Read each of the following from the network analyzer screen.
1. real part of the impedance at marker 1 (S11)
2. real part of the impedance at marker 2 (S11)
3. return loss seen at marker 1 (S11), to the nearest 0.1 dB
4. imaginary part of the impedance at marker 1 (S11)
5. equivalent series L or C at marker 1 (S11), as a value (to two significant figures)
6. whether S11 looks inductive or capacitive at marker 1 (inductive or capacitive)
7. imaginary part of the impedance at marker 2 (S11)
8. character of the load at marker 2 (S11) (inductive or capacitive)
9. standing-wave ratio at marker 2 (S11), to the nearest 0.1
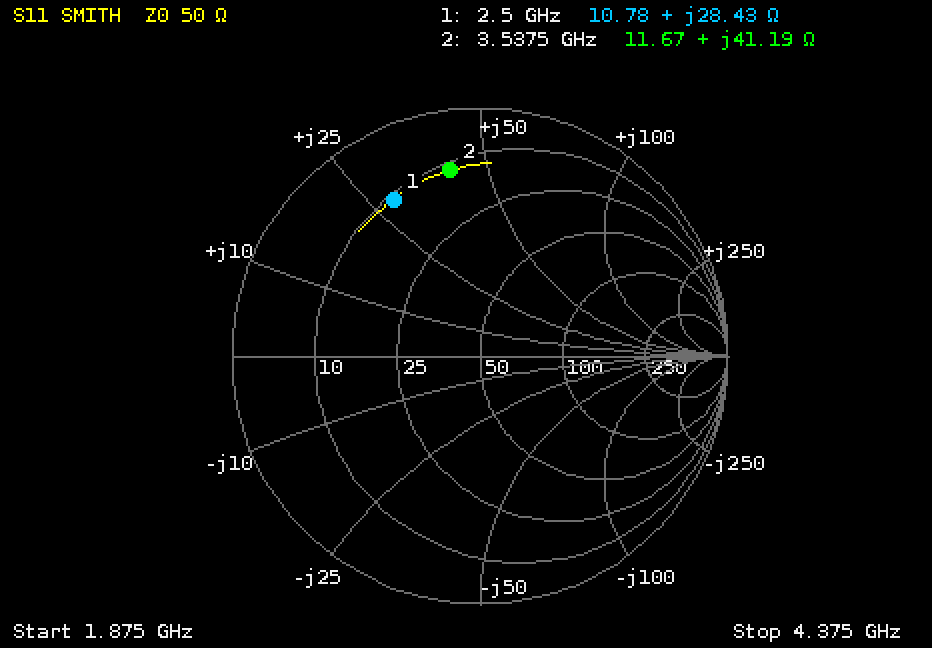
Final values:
10.78 Ω
11.67 Ω
2.8 dB
+28.43 Ω
1.8 nH
inductive
+41.19 Ω
inductive
7.3
